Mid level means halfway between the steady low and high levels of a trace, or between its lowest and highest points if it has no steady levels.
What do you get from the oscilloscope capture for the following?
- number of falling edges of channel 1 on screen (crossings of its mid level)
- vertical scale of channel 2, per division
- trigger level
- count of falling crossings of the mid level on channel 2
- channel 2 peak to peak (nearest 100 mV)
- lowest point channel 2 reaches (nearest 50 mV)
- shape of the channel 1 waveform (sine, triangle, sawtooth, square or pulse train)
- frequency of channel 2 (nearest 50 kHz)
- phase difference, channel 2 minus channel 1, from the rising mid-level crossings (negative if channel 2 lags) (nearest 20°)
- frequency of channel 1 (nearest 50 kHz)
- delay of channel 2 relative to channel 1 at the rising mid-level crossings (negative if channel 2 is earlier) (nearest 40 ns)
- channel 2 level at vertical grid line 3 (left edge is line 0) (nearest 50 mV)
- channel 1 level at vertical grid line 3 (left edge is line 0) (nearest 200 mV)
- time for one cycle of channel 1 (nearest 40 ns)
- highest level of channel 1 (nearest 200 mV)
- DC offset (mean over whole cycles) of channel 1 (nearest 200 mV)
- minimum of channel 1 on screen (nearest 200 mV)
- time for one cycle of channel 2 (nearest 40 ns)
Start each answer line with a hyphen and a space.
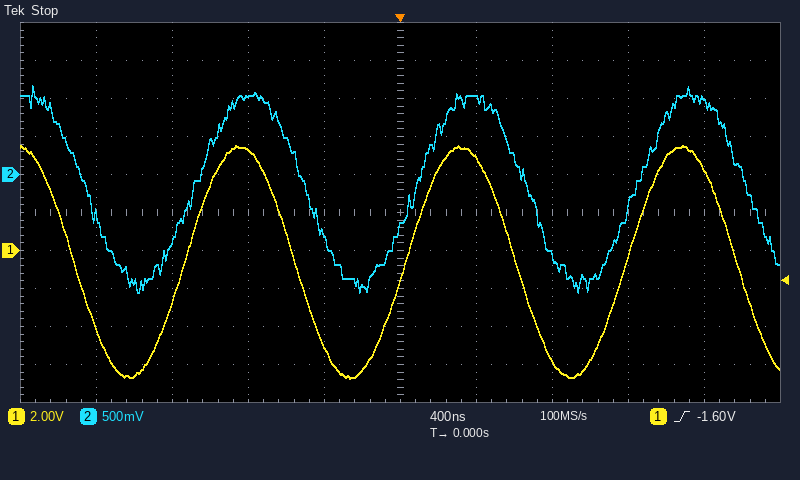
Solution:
- 4
- 500 mV
- -1.60 V
- 4
- 2.70 V
- -1.55 V
- sine
- 850 kHz
- -20°
- 850 kHz
- +40 ns
- 1.00 V
- 5.2 V
- 1.16 µs
- 5.6 V
- -600 mV
- -6.8 V
- 1.16 µs
